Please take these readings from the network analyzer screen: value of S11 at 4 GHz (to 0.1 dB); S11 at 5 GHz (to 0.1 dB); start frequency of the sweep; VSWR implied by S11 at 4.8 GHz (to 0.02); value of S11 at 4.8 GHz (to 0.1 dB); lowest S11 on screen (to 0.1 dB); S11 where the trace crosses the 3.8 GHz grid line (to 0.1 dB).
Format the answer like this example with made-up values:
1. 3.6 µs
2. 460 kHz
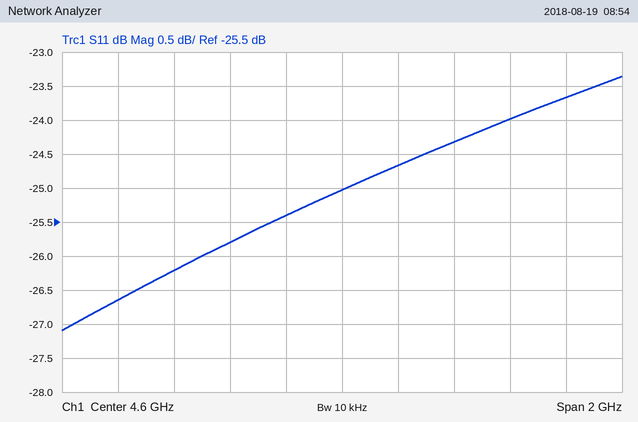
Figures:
1. -26.2 dB
2. -24.3 dB
3. 3.6 GHz
4. 1.12
5. -24.7 dB
6. -27.1 dB
7. -26.6 dB
